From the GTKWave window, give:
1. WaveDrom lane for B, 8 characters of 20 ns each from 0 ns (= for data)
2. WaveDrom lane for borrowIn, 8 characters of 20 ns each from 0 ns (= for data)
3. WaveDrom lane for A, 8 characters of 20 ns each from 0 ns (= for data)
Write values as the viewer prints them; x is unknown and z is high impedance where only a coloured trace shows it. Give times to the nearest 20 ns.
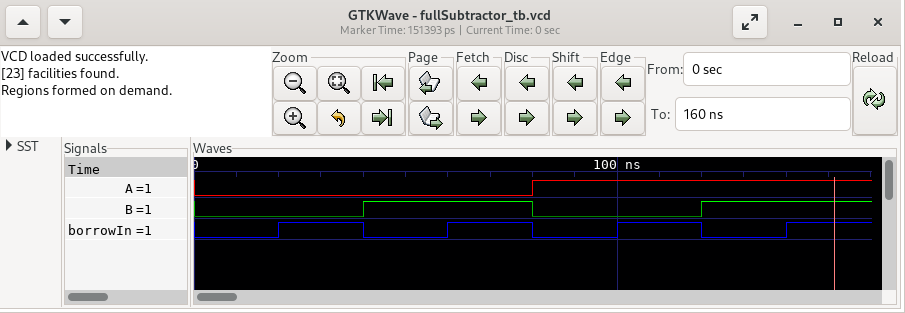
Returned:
{name: 'B', wave: '0.1.0.1.'}
{name: 'borrowIn', wave: '01010101'}
{name: 'A', wave: '0...1...'}
